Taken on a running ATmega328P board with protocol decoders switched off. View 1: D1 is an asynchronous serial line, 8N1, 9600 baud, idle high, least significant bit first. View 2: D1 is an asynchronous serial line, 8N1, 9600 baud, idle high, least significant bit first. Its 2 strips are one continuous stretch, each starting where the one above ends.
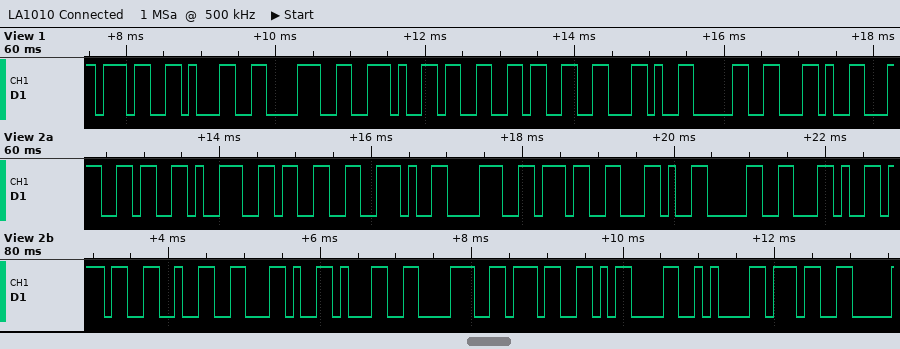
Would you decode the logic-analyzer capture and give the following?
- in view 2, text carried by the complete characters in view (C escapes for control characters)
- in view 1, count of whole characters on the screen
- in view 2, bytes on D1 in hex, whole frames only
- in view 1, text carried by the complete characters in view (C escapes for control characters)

"693.87,0,72,187\r\n7"
9
36 39 33 2E 38 37 2C 30 2C 37 32 2C 31 38 37 0D 0A 37
"718.33,0,"
